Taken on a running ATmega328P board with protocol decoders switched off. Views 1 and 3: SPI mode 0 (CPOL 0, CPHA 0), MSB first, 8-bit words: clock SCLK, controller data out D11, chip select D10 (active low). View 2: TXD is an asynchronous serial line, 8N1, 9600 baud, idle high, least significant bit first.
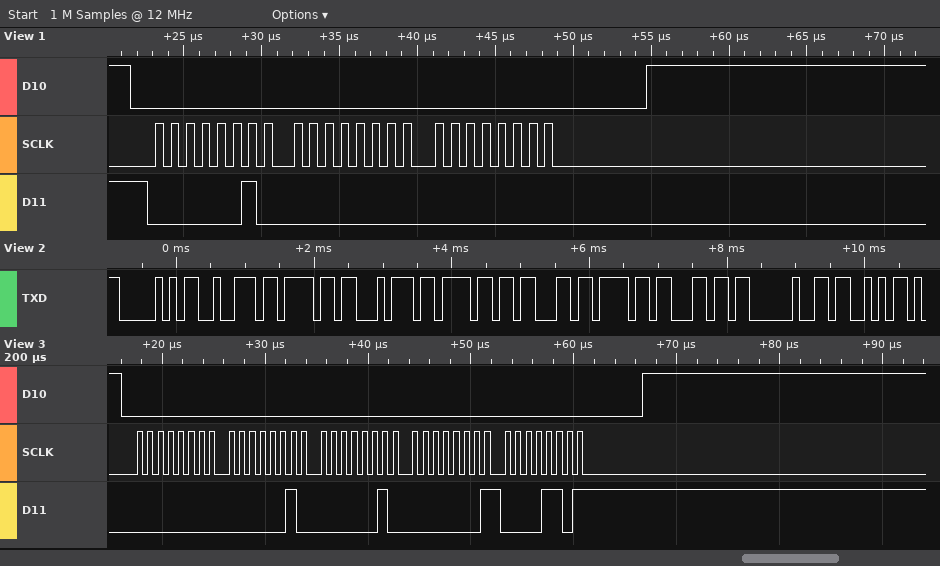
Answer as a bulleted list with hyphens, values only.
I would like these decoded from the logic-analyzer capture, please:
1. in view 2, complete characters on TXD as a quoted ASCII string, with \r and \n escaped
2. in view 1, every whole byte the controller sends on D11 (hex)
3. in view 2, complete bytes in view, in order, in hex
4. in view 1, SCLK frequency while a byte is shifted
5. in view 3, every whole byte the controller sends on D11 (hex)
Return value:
- "Protocol S"
- 02 00 00
- 50 72 6F 74 6F 63 6F 6C 20 53
- 1 MHz
- 00 02 02 01 0D
